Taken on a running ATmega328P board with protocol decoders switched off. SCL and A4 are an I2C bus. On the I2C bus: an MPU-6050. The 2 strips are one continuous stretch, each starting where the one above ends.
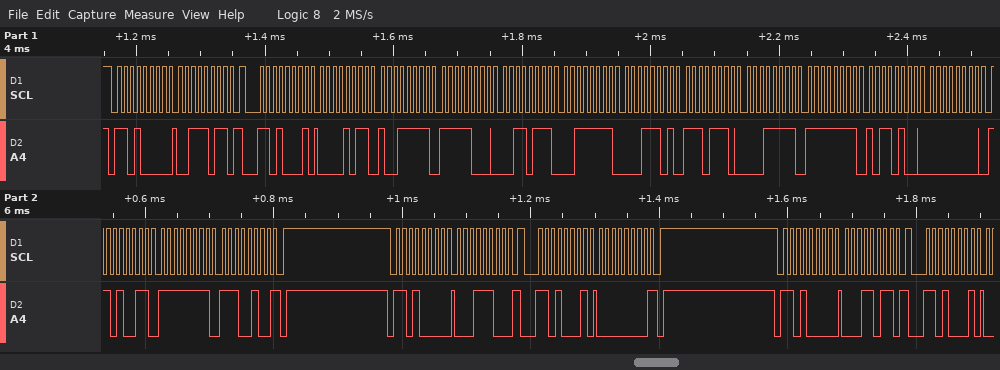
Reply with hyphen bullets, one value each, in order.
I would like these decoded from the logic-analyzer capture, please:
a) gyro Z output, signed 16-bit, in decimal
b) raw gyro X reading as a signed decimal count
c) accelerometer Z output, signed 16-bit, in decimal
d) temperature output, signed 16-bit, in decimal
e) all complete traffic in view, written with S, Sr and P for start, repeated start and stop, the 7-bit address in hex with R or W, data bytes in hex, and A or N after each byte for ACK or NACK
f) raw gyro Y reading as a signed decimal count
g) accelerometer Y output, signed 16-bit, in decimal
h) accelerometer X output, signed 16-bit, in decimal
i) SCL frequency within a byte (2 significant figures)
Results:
- -28
- -76
- 16157
- -4577
- S 68W A 3B A Sr 68R A 0B A 9F A F8 A 37 A 3F A 1D A EE A 1F A FF A B4 A 00 A D3 A FF A E4 N P S 68W A 1C A Sr 68R A 00 N P S 68W A 1B A Sr 68R A
- 211
- -1993
- 2975
- 100 kHz
